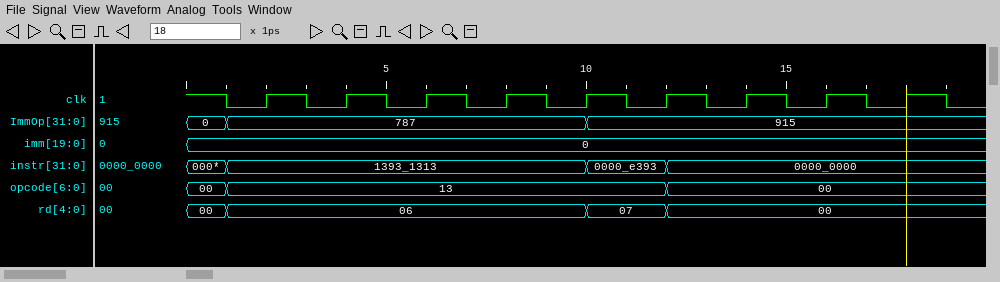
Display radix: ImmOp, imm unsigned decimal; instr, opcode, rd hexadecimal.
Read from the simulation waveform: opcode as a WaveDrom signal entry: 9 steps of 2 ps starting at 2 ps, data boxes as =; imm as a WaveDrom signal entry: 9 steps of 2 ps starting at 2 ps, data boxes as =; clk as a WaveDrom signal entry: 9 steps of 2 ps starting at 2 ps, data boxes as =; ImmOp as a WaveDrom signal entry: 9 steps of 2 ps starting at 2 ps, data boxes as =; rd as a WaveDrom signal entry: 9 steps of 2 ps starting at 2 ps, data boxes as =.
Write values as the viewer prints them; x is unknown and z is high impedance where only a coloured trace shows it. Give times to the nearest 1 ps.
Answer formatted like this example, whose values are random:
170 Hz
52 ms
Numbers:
{name: 'opcode', wave: '=....=...', data: '13 00'}
{name: 'imm', wave: '=........', data: '0'}
{name: 'clk', wave: 'p........'}
{name: 'ImmOp', wave: '=...=....', data: '787 915'}
{name: 'rd', wave: '=...==...', data: '06 07 00'}
